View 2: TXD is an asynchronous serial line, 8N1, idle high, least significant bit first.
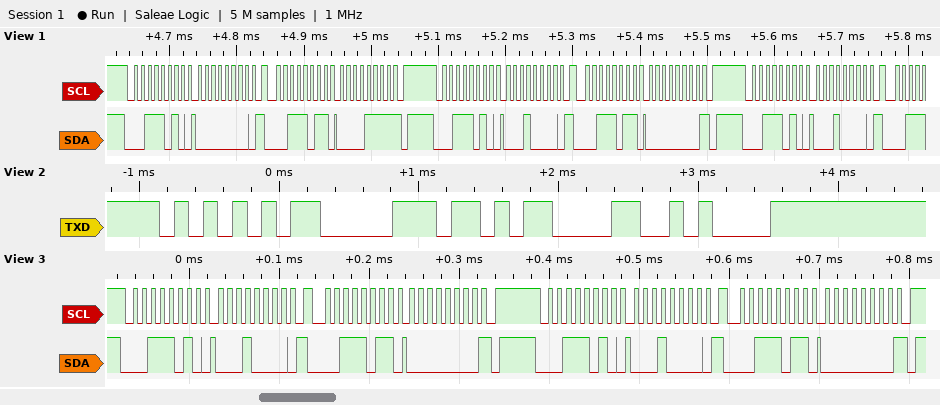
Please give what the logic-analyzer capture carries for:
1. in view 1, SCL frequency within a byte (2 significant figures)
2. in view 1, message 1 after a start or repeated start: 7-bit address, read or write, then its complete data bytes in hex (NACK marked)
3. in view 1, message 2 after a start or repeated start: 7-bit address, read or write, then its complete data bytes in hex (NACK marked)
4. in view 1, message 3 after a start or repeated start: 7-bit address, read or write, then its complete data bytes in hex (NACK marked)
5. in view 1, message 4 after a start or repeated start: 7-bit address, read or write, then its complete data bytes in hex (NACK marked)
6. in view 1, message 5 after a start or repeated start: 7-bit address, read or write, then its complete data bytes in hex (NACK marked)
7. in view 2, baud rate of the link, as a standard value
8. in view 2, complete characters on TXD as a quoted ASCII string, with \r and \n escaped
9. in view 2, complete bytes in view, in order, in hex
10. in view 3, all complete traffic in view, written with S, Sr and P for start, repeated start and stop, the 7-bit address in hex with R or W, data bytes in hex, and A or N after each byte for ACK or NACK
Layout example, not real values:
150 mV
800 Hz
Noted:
100 kHz
0x1D write: 00
0x1D read: 0F NACK
0x1D write: 10
0x1D read: 00 NACK
0x1D write: 10
9600 baud
"Up\r\n"
55 70 0D 0A
S 1DW A 10 A Sr 1DR A 00 N P S 1DW A 10 A Sr 1DR A 00 N P
